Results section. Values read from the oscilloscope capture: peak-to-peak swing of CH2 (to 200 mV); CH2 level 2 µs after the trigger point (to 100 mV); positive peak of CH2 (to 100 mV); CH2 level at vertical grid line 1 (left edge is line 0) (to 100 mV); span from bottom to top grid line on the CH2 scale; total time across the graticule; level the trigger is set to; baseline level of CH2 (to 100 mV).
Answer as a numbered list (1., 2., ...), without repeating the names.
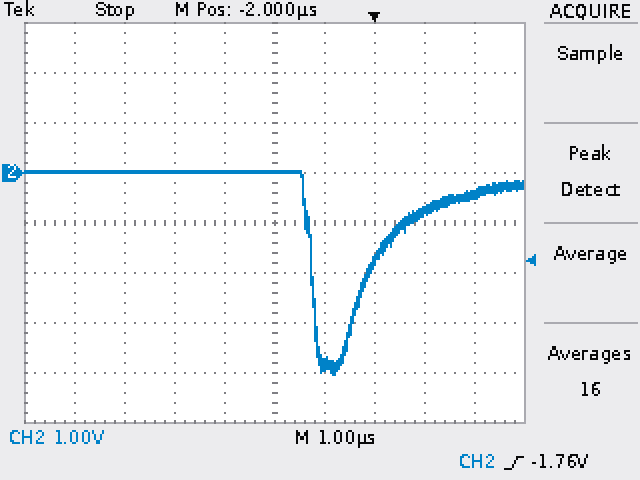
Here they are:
1. 4.0 V
2. -400 mV
3. 0.0 V
4. 0.0 V
5. 8 V
6. 10 µs
7. -1.76 V
8. 0.0 V
